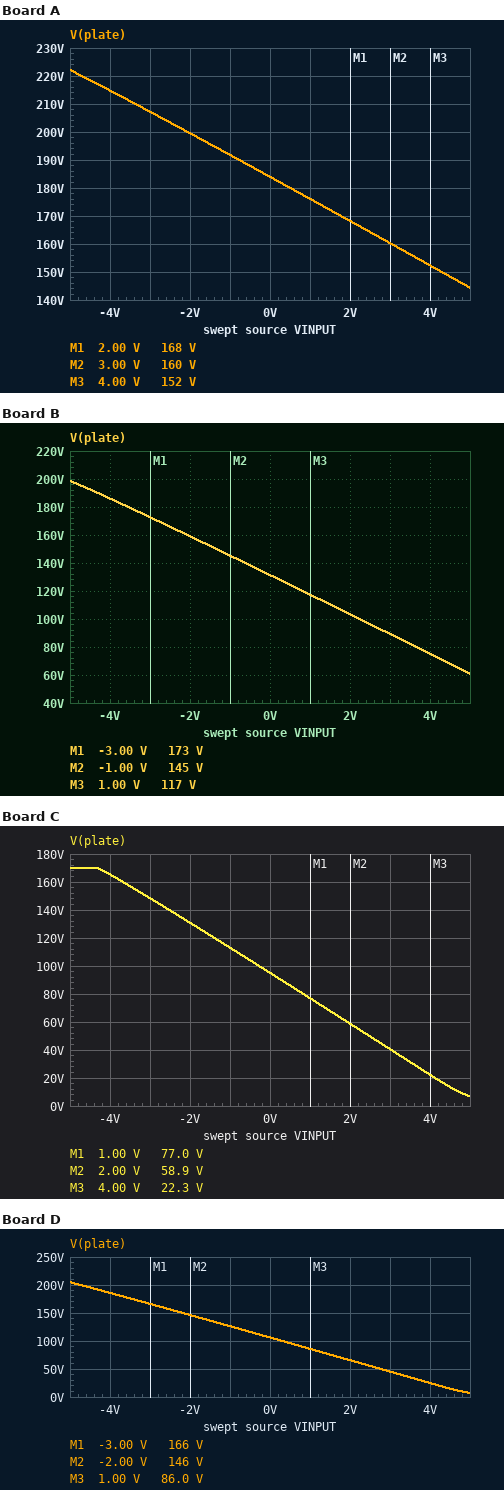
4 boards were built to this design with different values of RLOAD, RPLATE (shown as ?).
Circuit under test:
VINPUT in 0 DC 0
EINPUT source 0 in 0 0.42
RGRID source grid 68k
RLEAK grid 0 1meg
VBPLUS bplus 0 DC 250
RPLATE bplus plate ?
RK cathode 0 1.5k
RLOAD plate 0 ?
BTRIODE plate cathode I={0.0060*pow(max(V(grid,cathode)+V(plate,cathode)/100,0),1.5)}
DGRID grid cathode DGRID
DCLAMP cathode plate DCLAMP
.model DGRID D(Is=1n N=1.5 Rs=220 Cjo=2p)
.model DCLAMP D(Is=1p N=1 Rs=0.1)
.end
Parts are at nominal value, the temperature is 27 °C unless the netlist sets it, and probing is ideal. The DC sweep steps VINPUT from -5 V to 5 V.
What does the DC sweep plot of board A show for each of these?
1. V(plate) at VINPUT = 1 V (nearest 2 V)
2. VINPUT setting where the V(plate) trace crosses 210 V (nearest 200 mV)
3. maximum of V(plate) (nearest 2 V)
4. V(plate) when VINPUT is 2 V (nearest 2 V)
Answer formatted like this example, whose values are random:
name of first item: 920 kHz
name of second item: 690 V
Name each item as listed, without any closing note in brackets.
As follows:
V(plate) at VINPUT = 1 V: 176 V
VINPUT setting where the V(plate) trace crosses 210 V: -3.4 V
maximum of V(plate): 222 V
V(plate) when VINPUT is 2 V: 168 V
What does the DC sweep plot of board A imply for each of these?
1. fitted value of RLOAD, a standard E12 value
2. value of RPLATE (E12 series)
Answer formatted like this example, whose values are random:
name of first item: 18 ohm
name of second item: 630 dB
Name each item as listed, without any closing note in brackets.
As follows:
fitted value of RLOAD, a standard E12 value: 470 kΩ
value of RPLATE: 47 kΩ
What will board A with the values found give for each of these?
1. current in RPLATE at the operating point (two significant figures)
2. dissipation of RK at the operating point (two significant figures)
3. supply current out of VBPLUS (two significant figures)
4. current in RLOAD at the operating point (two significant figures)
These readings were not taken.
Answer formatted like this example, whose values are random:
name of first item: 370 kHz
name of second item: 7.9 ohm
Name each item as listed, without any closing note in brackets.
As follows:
current in RPLATE at the operating point: 1.4 mA
dissipation of RK at the operating point: 1.5 mW
supply current out of VBPLUS: 1.4 mA
current in RLOAD at the operating point: 390 µA
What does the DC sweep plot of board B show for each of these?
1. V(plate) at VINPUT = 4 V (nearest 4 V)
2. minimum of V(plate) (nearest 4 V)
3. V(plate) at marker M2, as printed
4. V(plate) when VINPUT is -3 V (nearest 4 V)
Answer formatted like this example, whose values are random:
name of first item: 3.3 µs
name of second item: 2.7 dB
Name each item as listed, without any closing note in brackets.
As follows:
V(plate) at VINPUT = 4 V: 76 V
minimum of V(plate): 60 V
V(plate) at marker M2, as printed: 145 V
V(plate) when VINPUT is -3 V: 172 V
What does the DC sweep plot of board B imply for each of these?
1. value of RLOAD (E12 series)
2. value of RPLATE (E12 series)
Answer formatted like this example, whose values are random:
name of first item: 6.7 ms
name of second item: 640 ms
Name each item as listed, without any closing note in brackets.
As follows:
value of RLOAD: 470 kΩ
value of RPLATE: 120 kΩ
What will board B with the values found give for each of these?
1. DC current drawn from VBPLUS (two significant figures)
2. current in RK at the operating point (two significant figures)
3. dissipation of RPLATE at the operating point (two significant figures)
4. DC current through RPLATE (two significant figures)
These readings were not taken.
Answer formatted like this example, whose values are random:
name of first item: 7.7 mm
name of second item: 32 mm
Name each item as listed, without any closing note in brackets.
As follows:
DC current drawn from VBPLUS: 990 µA
current in RK at the operating point: 710 µA
dissipation of RPLATE at the operating point: 120 mW
DC current through RPLATE: 990 µA
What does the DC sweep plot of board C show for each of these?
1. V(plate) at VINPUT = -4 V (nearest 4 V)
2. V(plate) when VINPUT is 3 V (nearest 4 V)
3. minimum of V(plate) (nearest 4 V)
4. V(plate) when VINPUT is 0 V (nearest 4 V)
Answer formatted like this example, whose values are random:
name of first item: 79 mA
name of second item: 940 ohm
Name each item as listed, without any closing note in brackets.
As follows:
V(plate) at VINPUT = -4 V: 164 V
V(plate) when VINPUT is 3 V: 40 V
minimum of V(plate): 8 V
V(plate) when VINPUT is 0 V: 96 V
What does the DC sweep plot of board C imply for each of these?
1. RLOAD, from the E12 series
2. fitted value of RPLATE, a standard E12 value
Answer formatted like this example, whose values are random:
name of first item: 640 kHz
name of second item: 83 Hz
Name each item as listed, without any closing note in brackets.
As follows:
RLOAD, from the E12 series: 470 kΩ
fitted value of RPLATE, a standard E12 value: 220 kΩ
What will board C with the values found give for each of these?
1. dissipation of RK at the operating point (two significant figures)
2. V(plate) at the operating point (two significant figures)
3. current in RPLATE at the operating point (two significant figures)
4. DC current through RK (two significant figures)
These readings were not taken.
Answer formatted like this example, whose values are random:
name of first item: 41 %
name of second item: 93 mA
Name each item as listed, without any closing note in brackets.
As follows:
dissipation of RK at the operating point: 380 µW
V(plate) at the operating point: 95 V
current in RPLATE at the operating point: 700 µA
DC current through RK: 500 µA
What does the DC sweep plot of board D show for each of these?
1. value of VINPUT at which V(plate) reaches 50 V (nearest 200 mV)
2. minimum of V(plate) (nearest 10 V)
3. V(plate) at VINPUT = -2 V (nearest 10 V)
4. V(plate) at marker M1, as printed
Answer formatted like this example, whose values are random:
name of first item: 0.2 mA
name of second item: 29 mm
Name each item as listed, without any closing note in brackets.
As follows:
value of VINPUT at which V(plate) reaches 50 V: 2.8 V
minimum of V(plate): 10 V
V(plate) at VINPUT = -2 V: 150 V
V(plate) at marker M1, as printed: 166 V
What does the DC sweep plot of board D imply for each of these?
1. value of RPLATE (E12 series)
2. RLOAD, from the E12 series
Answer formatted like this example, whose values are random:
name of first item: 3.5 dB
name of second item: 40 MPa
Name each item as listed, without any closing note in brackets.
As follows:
value of RPLATE: 220 kΩ
RLOAD, from the E12 series: 1.2 MΩ
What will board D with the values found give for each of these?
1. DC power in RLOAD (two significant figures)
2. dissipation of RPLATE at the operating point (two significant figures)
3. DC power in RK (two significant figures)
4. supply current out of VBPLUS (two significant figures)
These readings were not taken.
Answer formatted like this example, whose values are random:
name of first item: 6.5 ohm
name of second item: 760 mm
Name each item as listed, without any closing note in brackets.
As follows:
DC power in RLOAD: 9.4 mW
dissipation of RPLATE at the operating point: 94 mW
DC power in RK: 480 µW
supply current out of VBPLUS: 650 µA
